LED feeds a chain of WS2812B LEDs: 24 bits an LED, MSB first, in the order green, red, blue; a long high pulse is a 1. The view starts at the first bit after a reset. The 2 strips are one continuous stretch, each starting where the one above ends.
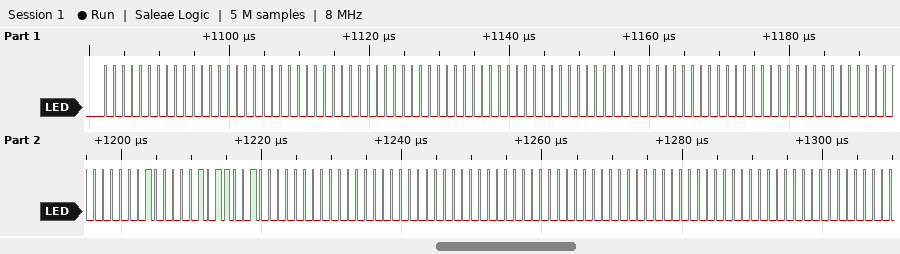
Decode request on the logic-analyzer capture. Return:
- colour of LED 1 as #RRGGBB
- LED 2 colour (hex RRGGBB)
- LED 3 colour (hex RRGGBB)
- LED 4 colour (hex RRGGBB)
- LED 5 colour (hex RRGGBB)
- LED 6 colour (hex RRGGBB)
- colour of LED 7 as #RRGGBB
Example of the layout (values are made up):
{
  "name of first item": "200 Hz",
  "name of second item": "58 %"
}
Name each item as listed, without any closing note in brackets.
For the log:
{
  "colour of LED 1 as #RRGGBB": "#000000",
  "LED 2 colour": "#000000",
  "LED 3 colour": "#000000",
  "LED 4 colour": "#000000",
  "LED 5 colour": "#644100",
  "LED 6 colour": "#000000",
  "colour of LED 7 as #RRGGBB": "#000000"
}
